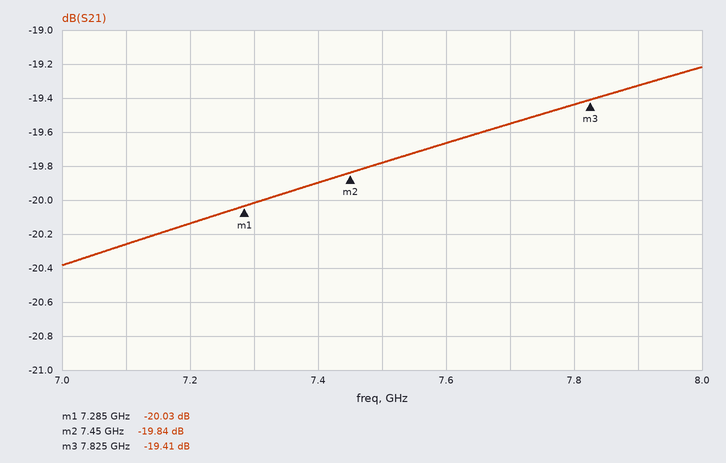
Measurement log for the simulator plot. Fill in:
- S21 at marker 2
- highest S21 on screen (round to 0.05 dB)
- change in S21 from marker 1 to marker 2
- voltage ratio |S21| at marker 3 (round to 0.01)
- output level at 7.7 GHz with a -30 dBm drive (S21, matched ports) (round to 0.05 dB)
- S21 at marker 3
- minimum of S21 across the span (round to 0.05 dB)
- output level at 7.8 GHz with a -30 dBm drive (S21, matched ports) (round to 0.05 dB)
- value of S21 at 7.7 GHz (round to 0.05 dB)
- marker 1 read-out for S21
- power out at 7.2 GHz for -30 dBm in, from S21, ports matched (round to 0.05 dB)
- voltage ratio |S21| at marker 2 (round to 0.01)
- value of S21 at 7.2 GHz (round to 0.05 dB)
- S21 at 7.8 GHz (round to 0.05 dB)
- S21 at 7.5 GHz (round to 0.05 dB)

-19.84 dB
-19.20 dB
0.19 dB
0.11
-49.55 dBm
-19.41 dB
-20.40 dB
-49.45 dBm
-19.55 dB
-20.03 dB
-50.15 dBm
0.10
-20.15 dB
-19.45 dB
-19.80 dB
